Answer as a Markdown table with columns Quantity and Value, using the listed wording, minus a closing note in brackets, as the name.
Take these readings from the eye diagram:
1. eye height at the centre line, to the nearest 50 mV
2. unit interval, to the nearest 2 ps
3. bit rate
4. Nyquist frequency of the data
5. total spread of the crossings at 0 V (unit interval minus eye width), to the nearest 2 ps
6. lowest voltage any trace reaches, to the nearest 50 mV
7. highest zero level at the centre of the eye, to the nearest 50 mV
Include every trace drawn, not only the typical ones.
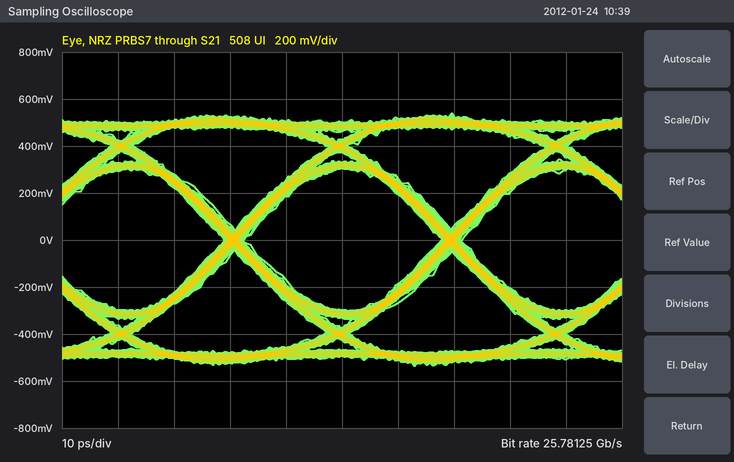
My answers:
| Quantity | Value |
|---|---|
| eye height at the centre line, to the nearest 50 mV | 600 mV |
| unit interval, to the nearest 2 ps | 38 ps |
| bit rate | 25.78125 Gb/s |
| Nyquist frequency of the data | 12.89062 GHz |
| total spread of the crossings at 0 V (unit interval minus eye width), to the nearest 2 ps | 4 ps |
| lowest voltage any trace reaches, to the nearest 50 mV | -550 mV |
| highest zero level at the centre of the eye, to the nearest 50 mV | -300 mV |
